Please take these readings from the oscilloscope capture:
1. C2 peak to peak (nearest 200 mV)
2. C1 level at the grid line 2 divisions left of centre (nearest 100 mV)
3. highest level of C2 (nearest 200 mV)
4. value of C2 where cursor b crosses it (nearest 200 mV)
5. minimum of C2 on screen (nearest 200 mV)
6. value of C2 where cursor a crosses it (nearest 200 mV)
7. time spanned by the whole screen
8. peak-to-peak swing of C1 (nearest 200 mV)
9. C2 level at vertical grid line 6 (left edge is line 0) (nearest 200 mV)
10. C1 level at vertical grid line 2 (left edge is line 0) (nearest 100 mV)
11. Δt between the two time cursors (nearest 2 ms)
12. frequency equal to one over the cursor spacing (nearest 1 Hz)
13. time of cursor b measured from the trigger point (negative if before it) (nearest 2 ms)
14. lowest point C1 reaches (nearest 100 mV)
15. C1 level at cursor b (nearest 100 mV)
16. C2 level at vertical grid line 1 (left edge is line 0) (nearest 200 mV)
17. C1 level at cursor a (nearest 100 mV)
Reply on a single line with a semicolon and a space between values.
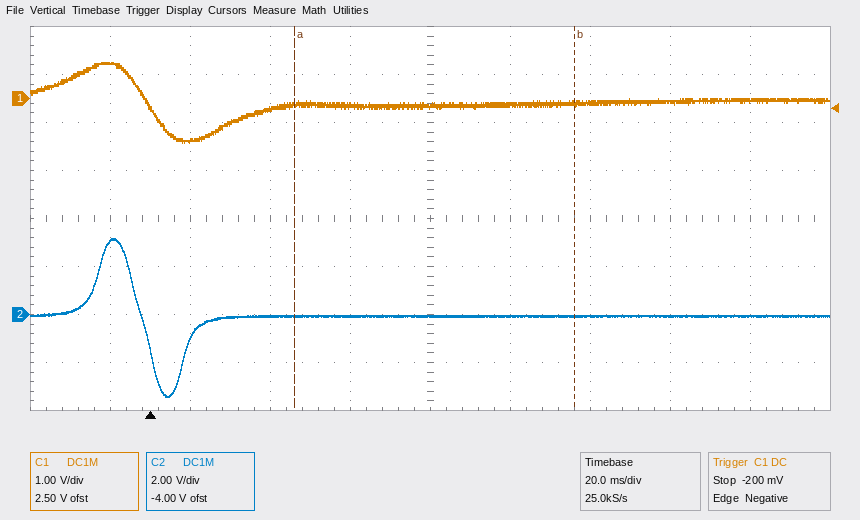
6.6 V; -200 mV; 3.2 V; 0.0 V; -3.4 V; 0.0 V; 200 ms; 1.6 V; 0.0 V; -900 mV; 70 ms; 14 Hz; +106 ms; -900 mV; -100 mV; 3.0 V; -100 mV
